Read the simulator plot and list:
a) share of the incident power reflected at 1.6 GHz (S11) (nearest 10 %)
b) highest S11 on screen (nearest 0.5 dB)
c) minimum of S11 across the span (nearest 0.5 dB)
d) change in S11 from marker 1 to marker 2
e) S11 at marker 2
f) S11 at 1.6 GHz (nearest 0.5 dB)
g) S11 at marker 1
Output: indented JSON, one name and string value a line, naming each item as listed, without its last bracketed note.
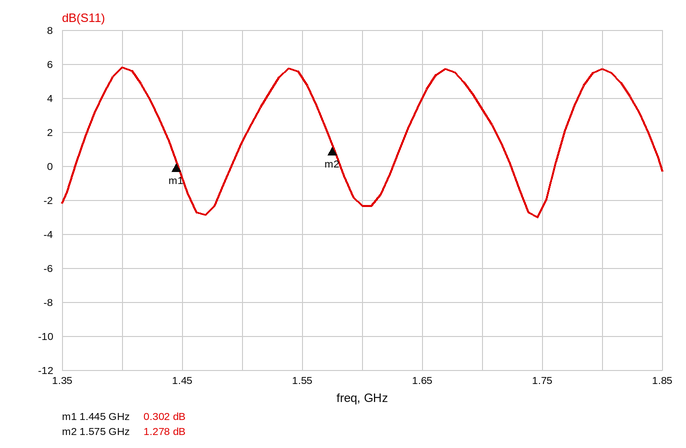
{
  "share of the incident power reflected at 1.6 GHz (S11)": "60 %",
  "highest S11 on screen": "6.0 dB",
  "minimum of S11 across the span": "-3.0 dB",
  "change in S11 from marker 1 to marker 2": "0.976 dB",
  "S11 at marker 2": "1.278 dB",
  "S11 at 1.6 GHz": "-2.5 dB",
  "S11 at marker 1": "0.302 dB"
}
